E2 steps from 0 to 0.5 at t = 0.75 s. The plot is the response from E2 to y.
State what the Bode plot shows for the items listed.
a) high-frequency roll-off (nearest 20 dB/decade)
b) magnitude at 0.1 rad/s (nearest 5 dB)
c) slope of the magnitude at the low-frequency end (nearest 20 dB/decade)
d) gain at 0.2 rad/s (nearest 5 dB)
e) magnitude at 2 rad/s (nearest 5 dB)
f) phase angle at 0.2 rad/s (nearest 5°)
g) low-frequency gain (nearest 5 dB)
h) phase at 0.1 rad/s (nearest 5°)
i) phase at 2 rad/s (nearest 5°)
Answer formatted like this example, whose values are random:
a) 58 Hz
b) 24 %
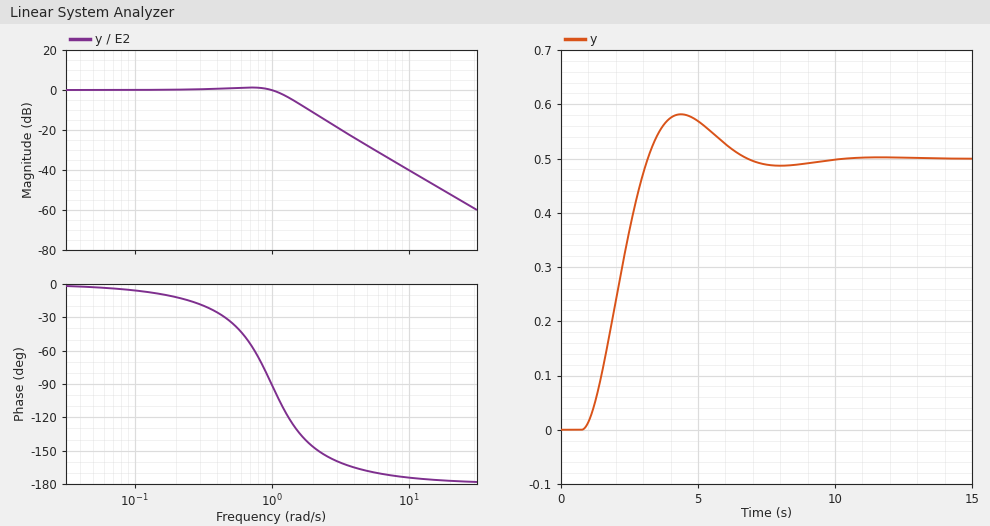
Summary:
a) -40 dB/decade
b) 0 dB
c) 0 dB/decade
d) 0 dB
e) -10 dB
f) -10°
g) 0 dB
h) -5°
i) -145°
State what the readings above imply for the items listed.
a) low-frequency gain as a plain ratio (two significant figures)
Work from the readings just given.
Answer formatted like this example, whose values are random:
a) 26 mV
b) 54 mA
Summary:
a) 1.0
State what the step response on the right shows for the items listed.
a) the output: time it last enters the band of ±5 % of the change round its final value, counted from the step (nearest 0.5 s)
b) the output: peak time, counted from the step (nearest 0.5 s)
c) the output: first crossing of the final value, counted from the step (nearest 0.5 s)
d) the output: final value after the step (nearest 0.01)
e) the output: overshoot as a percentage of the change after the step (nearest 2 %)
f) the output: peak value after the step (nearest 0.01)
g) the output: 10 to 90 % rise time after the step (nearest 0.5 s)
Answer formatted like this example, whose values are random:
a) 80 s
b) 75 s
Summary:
a) 5.5 s
b) 3.5 s
c) 2.5 s
d) 0.50
e) 16 %
f) 0.58
g) 1.5 s
